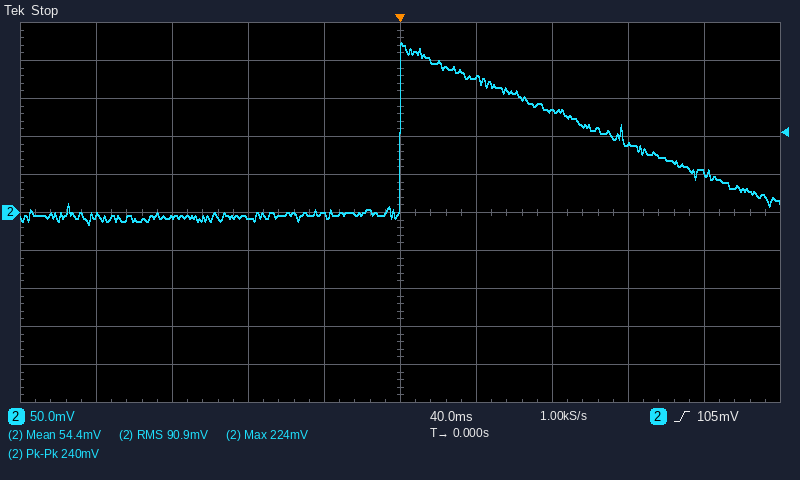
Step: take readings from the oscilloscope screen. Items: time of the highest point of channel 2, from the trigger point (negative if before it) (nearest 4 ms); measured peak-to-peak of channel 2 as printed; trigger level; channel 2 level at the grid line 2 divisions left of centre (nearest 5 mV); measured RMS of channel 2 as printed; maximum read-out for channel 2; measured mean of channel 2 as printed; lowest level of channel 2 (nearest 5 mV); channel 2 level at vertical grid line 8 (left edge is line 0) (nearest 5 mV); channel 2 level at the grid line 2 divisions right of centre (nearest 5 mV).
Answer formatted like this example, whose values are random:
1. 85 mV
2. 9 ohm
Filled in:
1. 0 ms
2. 240 mV
3. 105 mV
4. -5 mV
5. 90.9 mV
6. 224 mV
7. 54.4 mV
8. -15 mV
9. 90 mV
10. 135 mV
